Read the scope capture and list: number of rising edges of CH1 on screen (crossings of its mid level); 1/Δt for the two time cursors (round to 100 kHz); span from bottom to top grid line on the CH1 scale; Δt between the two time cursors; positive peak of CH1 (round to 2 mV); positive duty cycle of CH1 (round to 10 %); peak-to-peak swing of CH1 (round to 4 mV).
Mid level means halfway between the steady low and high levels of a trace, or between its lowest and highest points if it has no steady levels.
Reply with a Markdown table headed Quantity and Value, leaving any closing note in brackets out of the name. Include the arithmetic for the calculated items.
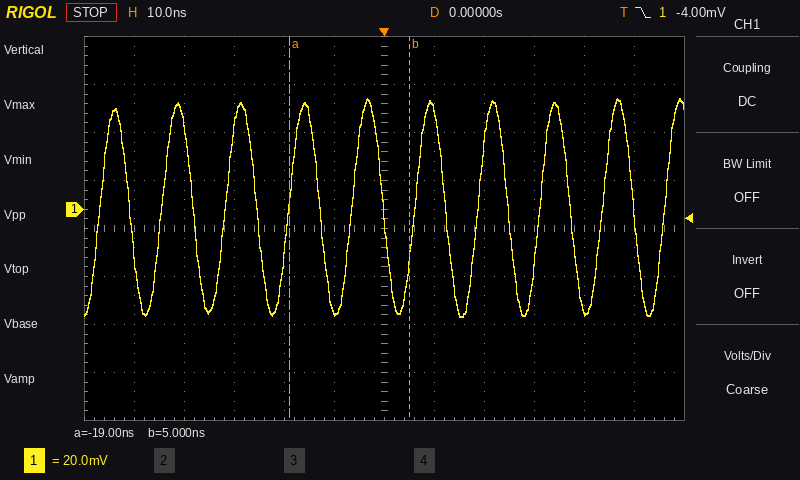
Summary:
| Quantity | Value |
|---|---|
| number of rising edges of CH1 on screen | 10 |
| 1/Δt for the two time cursors | 1 / 24 ns ≈ 41.7 MHz |
| span from bottom to top grid line on the CH1 scale | 160 mV |
| Δt between the two time cursors | 5 ns − (-19 ns) = 24 ns |
| positive peak of CH1 | 46 mV |
| positive duty cycle of CH1 | 50 % |
| peak-to-peak swing of CH1 | 92 mV |
